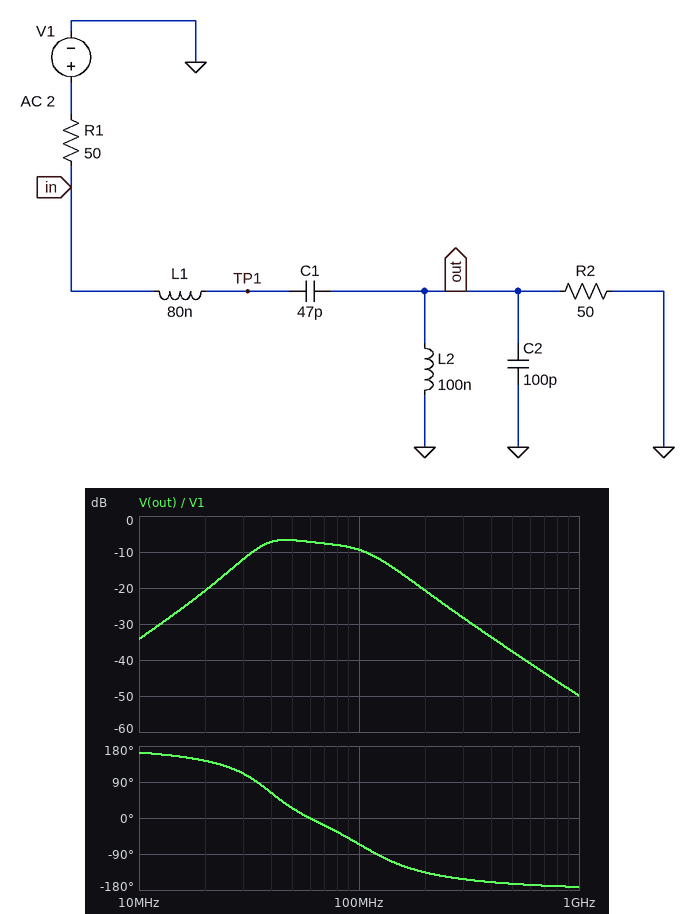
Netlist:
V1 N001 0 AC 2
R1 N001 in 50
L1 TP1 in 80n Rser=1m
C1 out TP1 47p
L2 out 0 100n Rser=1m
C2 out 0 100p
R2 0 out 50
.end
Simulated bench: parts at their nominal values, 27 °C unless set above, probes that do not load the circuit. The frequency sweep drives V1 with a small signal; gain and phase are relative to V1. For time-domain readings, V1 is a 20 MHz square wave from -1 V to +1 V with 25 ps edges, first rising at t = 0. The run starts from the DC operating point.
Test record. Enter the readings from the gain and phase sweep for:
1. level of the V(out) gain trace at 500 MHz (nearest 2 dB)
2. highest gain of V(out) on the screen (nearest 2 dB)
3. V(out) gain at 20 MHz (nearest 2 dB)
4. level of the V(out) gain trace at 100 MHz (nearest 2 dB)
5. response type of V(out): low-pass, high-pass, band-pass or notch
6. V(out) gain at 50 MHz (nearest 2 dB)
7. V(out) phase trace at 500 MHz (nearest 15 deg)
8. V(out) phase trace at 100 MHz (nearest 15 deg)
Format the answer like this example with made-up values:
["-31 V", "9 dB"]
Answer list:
["-38 dB", "-6 dB", "-20 dB", "-10 dB", "band-pass", "-6 dB", "-165 deg", "-60 deg"]
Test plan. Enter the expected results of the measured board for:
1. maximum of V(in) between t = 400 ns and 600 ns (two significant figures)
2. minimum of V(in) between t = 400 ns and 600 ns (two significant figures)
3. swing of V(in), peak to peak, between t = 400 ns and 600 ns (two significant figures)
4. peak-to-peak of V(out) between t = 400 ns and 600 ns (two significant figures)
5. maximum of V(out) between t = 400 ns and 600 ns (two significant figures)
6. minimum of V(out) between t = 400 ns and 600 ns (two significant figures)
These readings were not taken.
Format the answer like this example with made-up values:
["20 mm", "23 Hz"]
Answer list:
["1.1 V", "-1.1 V", "2.2 V", "670 mV", "330 mV", "-330 mV"]
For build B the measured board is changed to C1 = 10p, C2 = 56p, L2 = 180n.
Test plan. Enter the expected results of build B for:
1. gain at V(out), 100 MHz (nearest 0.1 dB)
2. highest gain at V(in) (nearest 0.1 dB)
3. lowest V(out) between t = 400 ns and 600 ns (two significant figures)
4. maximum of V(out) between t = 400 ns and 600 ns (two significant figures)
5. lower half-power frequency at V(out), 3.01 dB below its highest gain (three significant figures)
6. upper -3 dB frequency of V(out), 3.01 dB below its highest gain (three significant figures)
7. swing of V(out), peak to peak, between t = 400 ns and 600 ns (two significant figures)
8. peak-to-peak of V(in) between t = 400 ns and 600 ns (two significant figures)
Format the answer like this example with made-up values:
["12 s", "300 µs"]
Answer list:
["-13.9 dB", "0 dB", "-270 mV", "270 mV", "99.1 MHz", "229 MHz", "540 mV", "2.5 V"]
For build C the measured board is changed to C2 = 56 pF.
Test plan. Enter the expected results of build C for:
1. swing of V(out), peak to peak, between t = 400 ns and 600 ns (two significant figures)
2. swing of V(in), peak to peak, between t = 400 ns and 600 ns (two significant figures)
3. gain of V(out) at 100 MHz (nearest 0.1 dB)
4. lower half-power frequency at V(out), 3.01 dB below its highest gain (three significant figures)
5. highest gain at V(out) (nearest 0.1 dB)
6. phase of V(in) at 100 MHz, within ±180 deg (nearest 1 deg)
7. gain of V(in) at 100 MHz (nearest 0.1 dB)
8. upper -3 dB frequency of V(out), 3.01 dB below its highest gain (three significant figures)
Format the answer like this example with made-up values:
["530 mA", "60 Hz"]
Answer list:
["910 mV", "2.2 V", "-6.5 dB", "37.8 MHz", "-6.1 dB", "-12 deg", "-8.9 dB", "141 MHz"]
